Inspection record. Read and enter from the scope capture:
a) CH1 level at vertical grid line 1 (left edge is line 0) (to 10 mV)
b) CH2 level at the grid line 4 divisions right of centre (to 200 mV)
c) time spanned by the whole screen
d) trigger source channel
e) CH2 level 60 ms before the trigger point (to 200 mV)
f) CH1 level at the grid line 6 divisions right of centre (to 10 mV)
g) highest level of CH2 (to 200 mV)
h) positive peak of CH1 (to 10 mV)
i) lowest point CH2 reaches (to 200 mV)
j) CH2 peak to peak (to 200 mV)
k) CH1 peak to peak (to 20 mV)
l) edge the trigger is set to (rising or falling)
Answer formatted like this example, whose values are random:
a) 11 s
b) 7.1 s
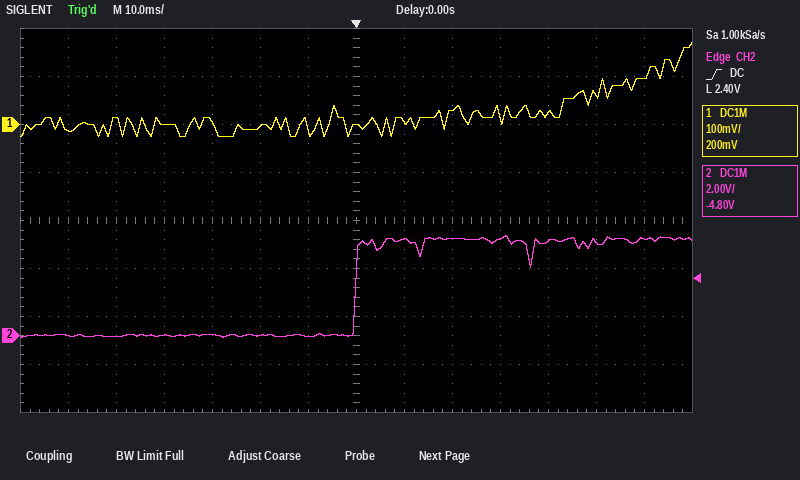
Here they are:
a) -10 mV
b) 4.0 V
c) 140 ms
d) CH2
e) 0.0 V
f) 100 mV
g) 4.2 V
h) 170 mV
i) 0.0 V
j) 4.2 V
k) 200 mV
l) rising
